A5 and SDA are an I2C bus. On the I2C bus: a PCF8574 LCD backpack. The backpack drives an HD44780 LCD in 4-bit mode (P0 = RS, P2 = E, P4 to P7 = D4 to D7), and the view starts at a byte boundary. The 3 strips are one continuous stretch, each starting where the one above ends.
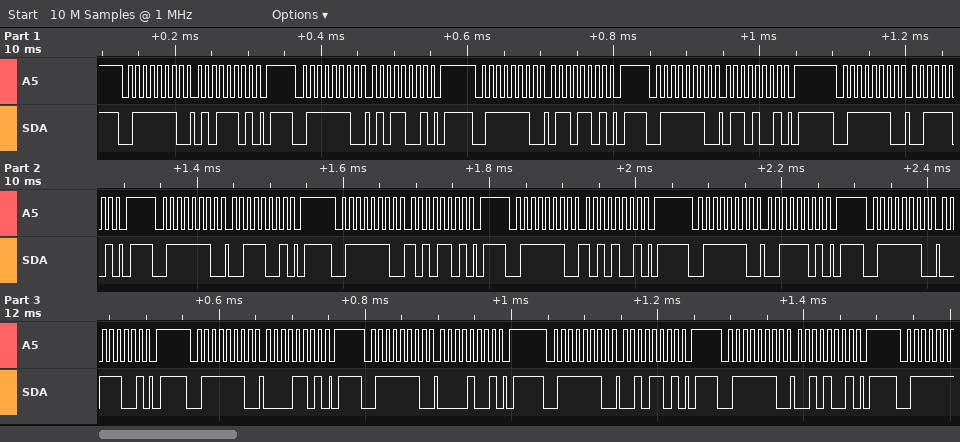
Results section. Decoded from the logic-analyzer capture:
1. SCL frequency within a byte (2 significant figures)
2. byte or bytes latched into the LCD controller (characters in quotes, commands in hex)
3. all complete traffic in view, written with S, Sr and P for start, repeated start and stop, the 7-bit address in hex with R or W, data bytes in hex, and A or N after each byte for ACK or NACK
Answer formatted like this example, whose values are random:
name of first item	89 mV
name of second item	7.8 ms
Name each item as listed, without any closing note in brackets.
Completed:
SCL frequency within a byte	100 kHz
byte or bytes latched into the LCD controller	'V' ':' '0'
all complete traffic in view, written with S, Sr and P for start, repeated start and stop, the 7-bit address in hex with R or W, data bytes in hex, and A or N after each byte for ACK or NACK	S 3FW A 5D A P S 3FW A 59 A P S 3FW A 6D A P S 3FW A 69 A P S 3FW A 3D A P S 3FW A 39 A P S 3FW A AD A P S 3FW A A9 A P S 3FW A 3D A P S 3FW A 39 A P S 3FW A 0D A P S 3FW A 09 A P S 3FW A 2D A P S 3FW A 29 A P
